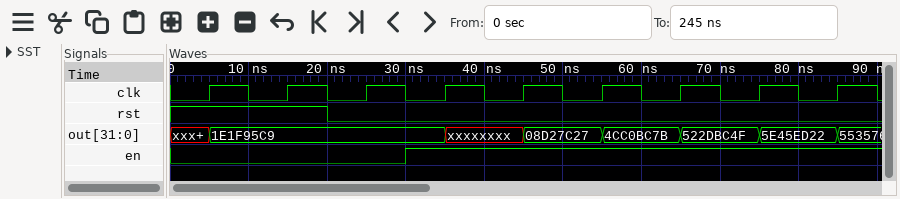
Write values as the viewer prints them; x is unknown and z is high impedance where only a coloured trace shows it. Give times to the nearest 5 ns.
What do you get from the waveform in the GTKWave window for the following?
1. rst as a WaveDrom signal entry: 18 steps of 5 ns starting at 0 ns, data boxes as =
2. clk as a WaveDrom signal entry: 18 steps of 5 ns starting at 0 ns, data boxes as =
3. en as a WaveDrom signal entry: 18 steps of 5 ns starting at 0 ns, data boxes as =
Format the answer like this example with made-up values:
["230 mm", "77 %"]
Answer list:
["{name: 'rst', wave: '1...0.............'}", "{name: 'clk', wave: '010101010101010101'}", "{name: 'en', wave: '0.....1...........'}"]
